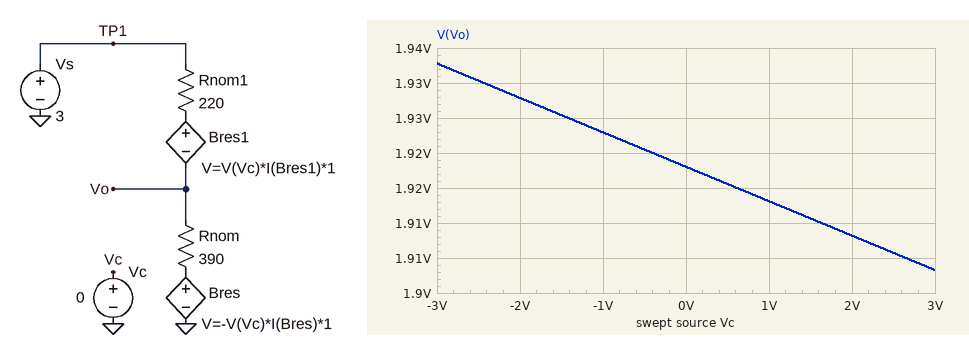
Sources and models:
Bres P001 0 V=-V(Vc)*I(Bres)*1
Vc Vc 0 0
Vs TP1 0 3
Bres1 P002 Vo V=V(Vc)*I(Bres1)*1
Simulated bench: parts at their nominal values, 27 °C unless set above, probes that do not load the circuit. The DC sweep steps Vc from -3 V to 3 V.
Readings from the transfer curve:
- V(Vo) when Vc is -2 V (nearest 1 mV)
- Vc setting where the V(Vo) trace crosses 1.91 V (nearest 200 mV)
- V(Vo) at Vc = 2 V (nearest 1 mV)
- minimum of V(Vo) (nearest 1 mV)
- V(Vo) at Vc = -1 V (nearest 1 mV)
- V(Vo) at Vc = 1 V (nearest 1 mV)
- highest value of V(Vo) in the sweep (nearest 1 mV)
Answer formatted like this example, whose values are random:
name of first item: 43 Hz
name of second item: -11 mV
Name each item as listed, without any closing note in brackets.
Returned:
V(Vo) when Vc is -2 V: 1.928 V
Vc setting where the V(Vo) trace crosses 1.91 V: 1.6 V
V(Vo) at Vc = 2 V: 1.908 V
minimum of V(Vo): 1.903 V
V(Vo) at Vc = -1 V: 1.923 V
V(Vo) at Vc = 1 V: 1.913 V
highest value of V(Vo) in the sweep: 1.933 V
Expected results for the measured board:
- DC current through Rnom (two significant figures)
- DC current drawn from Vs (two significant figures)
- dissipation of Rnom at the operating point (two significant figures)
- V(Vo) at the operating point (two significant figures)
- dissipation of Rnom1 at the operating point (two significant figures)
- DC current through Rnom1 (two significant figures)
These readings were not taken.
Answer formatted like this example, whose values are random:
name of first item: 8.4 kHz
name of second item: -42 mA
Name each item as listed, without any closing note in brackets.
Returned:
DC current through Rnom: 4.9 mA
DC current drawn from Vs: 4.9 mA
dissipation of Rnom at the operating point: 9.4 mW
V(Vo) at the operating point: 1.9 V
dissipation of Rnom1 at the operating point: 5.3 mW
DC current through Rnom1: 4.9 mA
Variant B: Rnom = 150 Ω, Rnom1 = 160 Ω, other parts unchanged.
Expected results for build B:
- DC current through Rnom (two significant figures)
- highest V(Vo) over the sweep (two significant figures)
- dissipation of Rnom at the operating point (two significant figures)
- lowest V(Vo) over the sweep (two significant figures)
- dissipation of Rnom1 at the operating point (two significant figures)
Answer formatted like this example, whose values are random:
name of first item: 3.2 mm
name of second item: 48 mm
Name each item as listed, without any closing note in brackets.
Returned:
DC current through Rnom: 9.7 mA
highest V(Vo) over the sweep: 1.5 V
dissipation of Rnom at the operating point: 14 mW
lowest V(Vo) over the sweep: 1.4 V
dissipation of Rnom1 at the operating point: 15 mW
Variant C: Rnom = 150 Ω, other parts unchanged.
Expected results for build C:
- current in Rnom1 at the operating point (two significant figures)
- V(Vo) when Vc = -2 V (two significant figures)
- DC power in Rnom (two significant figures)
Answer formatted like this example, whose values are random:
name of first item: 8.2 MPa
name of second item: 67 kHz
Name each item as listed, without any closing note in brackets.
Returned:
current in Rnom1 at the operating point: 8.1 mA
V(Vo) when Vc = -2 V: 1.2 V
DC power in Rnom: 9.9 mW
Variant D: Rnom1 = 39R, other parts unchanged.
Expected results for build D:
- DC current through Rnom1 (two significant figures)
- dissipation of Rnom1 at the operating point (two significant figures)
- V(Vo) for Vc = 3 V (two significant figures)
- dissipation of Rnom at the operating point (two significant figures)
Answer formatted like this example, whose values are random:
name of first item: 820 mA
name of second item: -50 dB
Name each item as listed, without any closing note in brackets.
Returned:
DC current through Rnom1: 7.0 mA
dissipation of Rnom1 at the operating point: 1.9 mW
V(Vo) for Vc = 3 V: 2.7 V
dissipation of Rnom at the operating point: 19 mW
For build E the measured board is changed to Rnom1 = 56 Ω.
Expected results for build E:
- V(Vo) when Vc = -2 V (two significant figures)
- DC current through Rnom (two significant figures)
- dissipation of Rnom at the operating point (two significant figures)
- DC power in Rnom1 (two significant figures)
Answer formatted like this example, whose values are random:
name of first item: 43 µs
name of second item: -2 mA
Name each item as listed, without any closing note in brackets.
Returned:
V(Vo) when Vc = -2 V: 2.6 V
DC current through Rnom: 6.7 mA
dissipation of Rnom at the operating point: 18 mW
DC power in Rnom1: 2.5 mW
